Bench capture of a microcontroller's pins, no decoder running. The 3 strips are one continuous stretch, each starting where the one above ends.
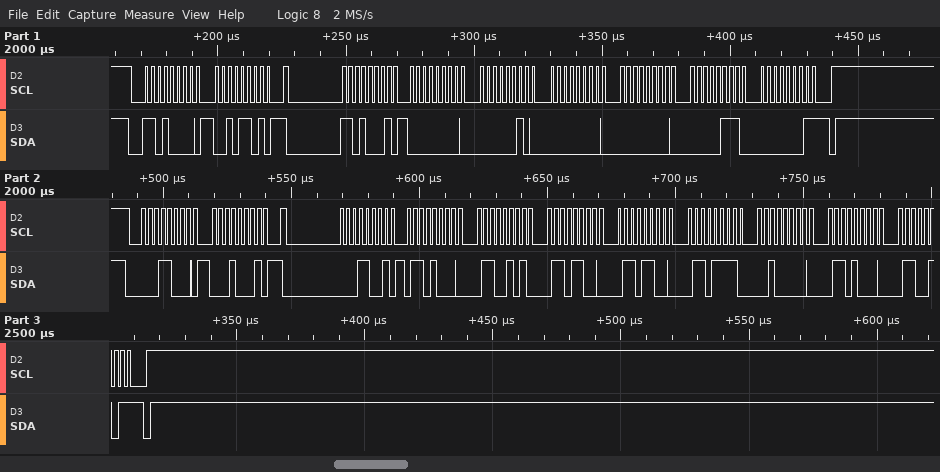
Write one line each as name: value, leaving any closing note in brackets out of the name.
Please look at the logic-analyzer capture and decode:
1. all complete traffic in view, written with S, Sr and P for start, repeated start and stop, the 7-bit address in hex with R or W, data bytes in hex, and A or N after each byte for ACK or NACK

all complete traffic in view, written with S, Sr and P for start, repeated start and stop, the 7-bit address in hex with R or W, data bytes in hex, and A or N after each byte for ACK or NACK: S 68W A 2D A Sr 68R A 00 A 02 A 00 A 00 A 07 A 01 N P S 0CW A 11 A Sr 0CR A 68 A 65 A 6C A 6C A 6F A 20 A 68 A 65 N P
